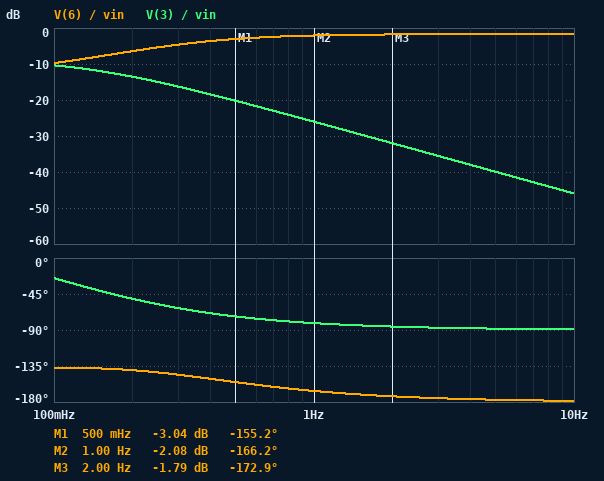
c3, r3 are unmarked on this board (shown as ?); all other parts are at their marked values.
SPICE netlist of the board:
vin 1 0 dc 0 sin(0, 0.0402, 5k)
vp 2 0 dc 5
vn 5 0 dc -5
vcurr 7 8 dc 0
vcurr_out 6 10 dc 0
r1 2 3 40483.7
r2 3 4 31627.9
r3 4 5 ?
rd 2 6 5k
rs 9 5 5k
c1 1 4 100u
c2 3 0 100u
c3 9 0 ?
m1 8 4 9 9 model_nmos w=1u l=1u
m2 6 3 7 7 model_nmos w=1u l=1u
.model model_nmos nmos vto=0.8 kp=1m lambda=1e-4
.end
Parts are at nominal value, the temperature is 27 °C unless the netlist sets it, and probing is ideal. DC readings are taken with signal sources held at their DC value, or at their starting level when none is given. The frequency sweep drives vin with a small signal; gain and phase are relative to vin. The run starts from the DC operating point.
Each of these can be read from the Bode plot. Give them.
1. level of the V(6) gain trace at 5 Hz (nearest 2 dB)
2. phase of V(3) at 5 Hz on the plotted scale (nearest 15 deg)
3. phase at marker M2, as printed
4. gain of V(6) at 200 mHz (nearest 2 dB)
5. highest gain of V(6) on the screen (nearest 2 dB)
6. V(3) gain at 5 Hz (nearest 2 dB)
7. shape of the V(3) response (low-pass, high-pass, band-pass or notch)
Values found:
-2 dB
-90 deg
-166.2 deg
-6 dB
-2 dB
-40 dB
low-pass
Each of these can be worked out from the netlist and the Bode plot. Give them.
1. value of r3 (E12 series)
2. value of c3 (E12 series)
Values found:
150 kΩ
270 µF
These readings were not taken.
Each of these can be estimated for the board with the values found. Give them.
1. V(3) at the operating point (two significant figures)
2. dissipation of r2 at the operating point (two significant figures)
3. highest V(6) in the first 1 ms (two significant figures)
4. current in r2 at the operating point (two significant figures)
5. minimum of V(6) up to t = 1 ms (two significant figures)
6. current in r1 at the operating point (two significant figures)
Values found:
3.2 V
64 µW
630 mV
45 µA
560 mV
45 µA
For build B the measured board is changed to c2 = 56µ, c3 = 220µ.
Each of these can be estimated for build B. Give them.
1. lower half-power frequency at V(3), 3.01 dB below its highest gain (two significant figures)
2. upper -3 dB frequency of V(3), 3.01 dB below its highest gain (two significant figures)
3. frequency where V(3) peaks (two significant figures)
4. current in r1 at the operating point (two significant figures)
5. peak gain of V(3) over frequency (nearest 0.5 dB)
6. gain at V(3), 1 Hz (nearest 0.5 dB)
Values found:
22 mHz
240 mHz
72 mHz
45 µA
-8.0 dB
-21.0 dB
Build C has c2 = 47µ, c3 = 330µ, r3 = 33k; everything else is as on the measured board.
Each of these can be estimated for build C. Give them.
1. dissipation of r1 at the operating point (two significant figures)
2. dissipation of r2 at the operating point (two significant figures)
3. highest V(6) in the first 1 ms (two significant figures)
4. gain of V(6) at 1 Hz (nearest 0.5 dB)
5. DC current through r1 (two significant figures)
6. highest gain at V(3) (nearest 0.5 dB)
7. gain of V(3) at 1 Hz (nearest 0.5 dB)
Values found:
370 µW
290 µW
3.6 V
11.0 dB
95 µA
-8.5 dB
-19.5 dB
